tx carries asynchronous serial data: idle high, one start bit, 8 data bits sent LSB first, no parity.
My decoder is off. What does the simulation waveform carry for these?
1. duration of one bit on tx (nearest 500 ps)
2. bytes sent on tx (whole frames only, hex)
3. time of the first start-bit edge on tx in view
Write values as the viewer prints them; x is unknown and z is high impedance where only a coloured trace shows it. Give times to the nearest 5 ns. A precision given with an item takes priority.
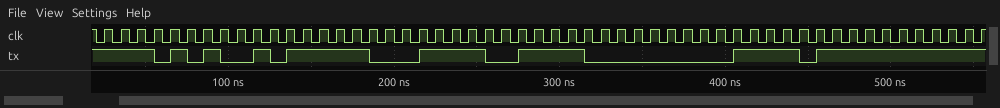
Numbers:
10000 ps
A5, 3C, 00, FF
55 ns
